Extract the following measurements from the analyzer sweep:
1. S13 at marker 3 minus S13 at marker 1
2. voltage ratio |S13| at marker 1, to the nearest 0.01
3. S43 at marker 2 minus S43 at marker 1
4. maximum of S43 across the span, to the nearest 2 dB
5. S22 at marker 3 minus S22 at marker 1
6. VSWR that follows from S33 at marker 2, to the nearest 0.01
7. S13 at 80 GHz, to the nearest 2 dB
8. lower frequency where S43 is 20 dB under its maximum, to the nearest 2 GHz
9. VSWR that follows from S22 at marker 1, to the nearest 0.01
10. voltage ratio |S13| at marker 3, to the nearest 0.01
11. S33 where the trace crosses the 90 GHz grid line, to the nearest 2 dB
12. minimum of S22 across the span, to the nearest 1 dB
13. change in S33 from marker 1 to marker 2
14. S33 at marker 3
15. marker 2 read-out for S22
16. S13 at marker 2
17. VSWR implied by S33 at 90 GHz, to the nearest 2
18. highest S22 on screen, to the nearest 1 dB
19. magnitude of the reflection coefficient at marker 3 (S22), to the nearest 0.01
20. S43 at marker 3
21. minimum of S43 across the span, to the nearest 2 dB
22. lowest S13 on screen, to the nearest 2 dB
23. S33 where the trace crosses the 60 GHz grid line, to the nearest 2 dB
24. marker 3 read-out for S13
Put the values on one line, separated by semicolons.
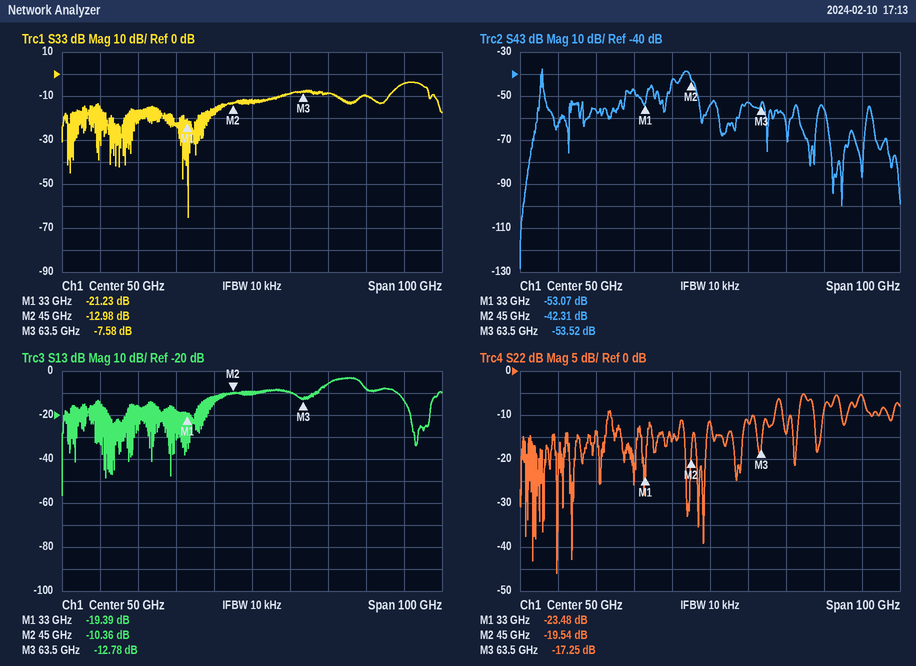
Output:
6.61 dB; 0.11; 10.76 dB; -38 dB; 6.23 dB; 1.58; -8 dB; 4 GHz; 1.14; 0.23; -4 dB; -46 dB; 8.25 dB; -7.58 dB; -19.54 dB; -10.36 dB; 4; -5 dB; 0.14; -53.52 dB; -128 dB; -56 dB; -8 dB; -12.78 dB
